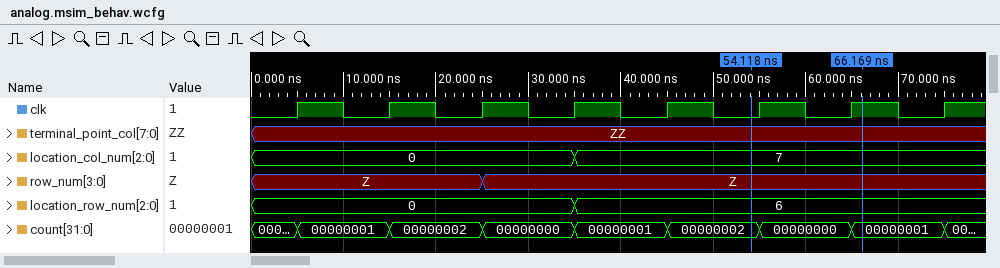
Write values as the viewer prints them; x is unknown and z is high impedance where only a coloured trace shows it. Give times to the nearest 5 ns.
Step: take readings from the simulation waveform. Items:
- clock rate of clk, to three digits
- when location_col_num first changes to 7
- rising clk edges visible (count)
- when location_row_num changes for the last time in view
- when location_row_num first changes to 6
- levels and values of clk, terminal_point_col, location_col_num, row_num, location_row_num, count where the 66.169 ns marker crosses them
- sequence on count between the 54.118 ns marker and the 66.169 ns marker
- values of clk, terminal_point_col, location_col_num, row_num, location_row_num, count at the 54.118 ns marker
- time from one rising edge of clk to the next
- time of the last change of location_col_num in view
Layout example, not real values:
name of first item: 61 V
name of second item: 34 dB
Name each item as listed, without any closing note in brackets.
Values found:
clock rate of clk, to three digits: 100 MHz
when location_col_num first changes to 7: 35 ns
rising clk edges visible: 8
when location_row_num changes for the last time in view: 35 ns
when location_row_num first changes to 6: 35 ns
levels and values of clk, terminal_point_col, location_col_num, row_num, location_row_num, count where the 66.169 ns marker crosses them: clk=1, terminal_point_col=ZZ, location_col_num=7, row_num=Z, location_row_num=6, count=00000001
sequence on count between the 54.118 ns marker and the 66.169 ns marker: 00000002, 00000000, 00000001
values of clk, terminal_point_col, location_col_num, row_num, location_row_num, count at the 54.118 ns marker: clk=0, terminal_point_col=ZZ, location_col_num=7, row_num=Z, location_row_num=6, count=00000002
time from one rising edge of clk to the next: 10 ns
time of the last change of location_col_num in view: 35 ns
